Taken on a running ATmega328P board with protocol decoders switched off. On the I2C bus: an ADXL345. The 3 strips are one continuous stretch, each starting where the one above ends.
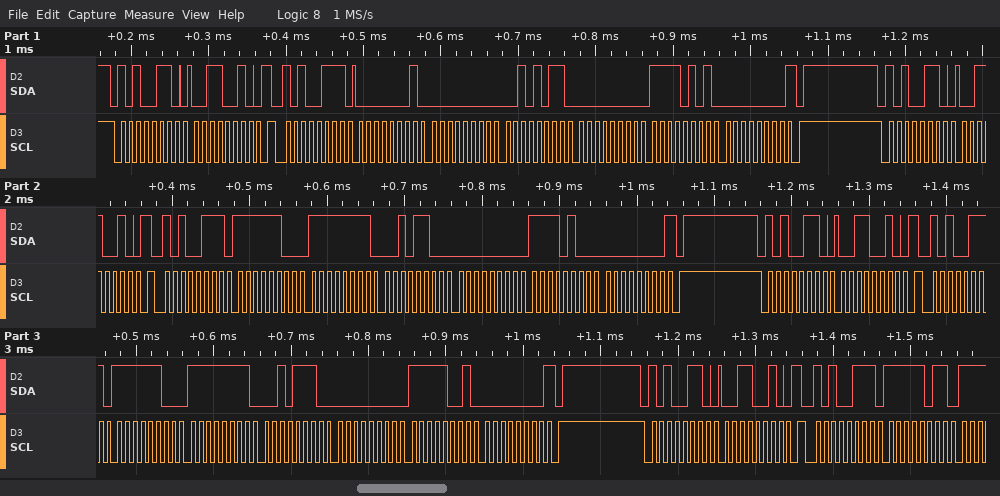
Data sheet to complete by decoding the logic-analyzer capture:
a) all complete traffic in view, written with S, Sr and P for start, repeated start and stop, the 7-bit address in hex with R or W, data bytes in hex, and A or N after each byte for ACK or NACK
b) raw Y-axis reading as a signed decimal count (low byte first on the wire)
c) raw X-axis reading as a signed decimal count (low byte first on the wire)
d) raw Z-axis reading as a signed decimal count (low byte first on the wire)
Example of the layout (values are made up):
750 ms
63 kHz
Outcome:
S 53W A 32 A Sr 53R A 01 A 00 A 2B A 00 A F5 A 00 N P S 53W A 32 A Sr 53R A FC A FF A 2C A 00 A F4 A 00 N P S 53W A 32 A Sr 53R A FC A FF A 2E A 00 A F9 A 00 N P S 53W A 32 A Sr 53R A FB A
43
1
245
